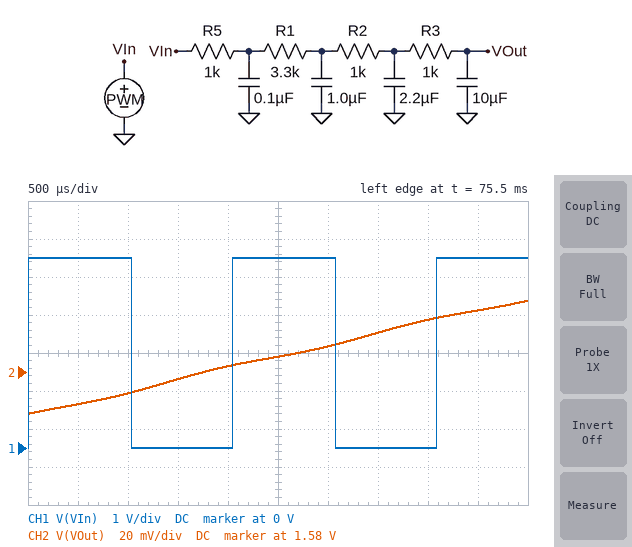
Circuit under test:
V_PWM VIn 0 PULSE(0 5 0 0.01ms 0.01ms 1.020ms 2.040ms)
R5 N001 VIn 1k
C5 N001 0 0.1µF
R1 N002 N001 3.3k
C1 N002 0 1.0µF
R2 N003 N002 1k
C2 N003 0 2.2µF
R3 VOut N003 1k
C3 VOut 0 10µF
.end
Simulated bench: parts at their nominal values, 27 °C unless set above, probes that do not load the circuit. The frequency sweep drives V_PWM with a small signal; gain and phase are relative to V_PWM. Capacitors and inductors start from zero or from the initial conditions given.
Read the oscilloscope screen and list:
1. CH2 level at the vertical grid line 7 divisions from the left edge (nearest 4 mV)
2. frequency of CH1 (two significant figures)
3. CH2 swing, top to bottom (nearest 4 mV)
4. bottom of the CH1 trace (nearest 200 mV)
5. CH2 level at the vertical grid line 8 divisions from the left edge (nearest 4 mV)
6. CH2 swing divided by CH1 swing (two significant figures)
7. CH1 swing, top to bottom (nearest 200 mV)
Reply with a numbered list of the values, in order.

1. 1.600 V
2. 490 Hz
3. 60 mV
4. 0 V
5. 1.608 V
6. 0.012
7. 5.0 V
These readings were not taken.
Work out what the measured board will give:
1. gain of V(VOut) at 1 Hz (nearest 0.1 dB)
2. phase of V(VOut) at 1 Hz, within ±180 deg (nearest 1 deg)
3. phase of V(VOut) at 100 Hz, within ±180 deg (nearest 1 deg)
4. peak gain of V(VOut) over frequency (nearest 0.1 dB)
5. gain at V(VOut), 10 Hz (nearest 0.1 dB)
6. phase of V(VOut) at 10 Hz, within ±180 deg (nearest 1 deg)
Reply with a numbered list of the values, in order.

1. -0.9 dB
2. -27 deg
3. -165 deg
4. 0 dB
5. -13.9 dB
6. -88 deg
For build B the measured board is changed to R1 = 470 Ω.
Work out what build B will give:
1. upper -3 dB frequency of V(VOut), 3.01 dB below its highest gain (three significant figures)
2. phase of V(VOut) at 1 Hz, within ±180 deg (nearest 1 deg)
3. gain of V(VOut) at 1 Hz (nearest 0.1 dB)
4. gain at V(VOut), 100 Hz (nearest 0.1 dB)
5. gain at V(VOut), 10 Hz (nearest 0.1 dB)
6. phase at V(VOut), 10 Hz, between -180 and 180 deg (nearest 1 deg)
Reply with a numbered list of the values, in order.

1. 4.03 Hz
2. -15 deg
3. -0.3 dB
4. -31.7 dB
5. -8.6 dB
6. -76 deg
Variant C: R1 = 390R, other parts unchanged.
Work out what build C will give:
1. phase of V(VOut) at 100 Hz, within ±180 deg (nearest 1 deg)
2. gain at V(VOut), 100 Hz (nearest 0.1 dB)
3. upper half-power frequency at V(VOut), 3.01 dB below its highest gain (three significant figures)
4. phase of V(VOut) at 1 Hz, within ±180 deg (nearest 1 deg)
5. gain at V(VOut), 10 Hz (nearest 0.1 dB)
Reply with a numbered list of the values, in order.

1. -153 deg
2. -31.4 dB
3. 4.13 Hz
4. -14 deg
5. -8.4 dB
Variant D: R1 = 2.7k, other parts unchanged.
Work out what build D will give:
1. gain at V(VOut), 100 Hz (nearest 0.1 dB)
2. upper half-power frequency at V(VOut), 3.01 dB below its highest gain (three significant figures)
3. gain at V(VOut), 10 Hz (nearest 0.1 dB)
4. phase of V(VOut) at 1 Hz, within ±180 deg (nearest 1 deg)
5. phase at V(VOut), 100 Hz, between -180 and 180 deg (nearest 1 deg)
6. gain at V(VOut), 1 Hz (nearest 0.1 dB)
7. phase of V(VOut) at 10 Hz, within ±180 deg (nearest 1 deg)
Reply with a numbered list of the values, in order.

1. -37.7 dB
2. 2.33 Hz
3. -13.0 dB
4. -24 deg
5. -164 deg
6. -0.7 dB
7. -87 deg
